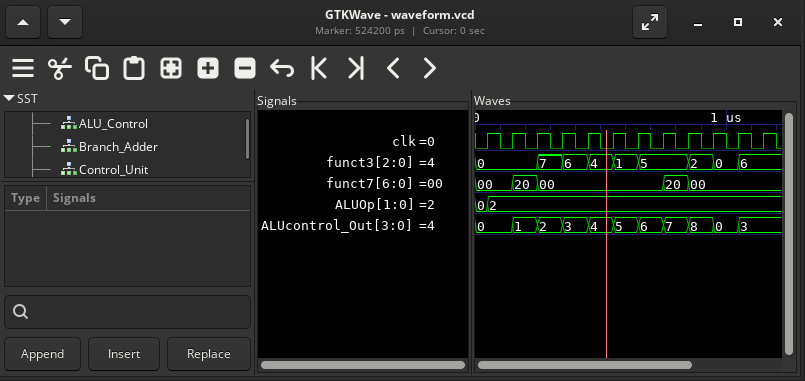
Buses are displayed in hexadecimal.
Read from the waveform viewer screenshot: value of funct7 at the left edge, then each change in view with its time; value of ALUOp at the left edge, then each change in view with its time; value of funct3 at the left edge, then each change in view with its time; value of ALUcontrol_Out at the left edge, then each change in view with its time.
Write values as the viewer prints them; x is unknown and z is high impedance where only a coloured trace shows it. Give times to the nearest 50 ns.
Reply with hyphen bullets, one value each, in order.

- 00, 20 at 150 ns, 00 at 250 ns, 20 at 750 ns, 00 at 850 ns
- 0, 2 at 50 ns
- 0, 7 at 250 ns, 6 at 350 ns, 4 at 450 ns, 1 at 550 ns, 5 at 650 ns, 2 at 850 ns, 0 at 950 ns, 6 at 1050 ns
- 0, 1 at 150 ns, 2 at 250 ns, 3 at 350 ns, 4 at 450 ns, 5 at 550 ns, 6 at 650 ns, 7 at 750 ns, 8 at 850 ns, 0 at 950 ns, 3 at 1050 ns
